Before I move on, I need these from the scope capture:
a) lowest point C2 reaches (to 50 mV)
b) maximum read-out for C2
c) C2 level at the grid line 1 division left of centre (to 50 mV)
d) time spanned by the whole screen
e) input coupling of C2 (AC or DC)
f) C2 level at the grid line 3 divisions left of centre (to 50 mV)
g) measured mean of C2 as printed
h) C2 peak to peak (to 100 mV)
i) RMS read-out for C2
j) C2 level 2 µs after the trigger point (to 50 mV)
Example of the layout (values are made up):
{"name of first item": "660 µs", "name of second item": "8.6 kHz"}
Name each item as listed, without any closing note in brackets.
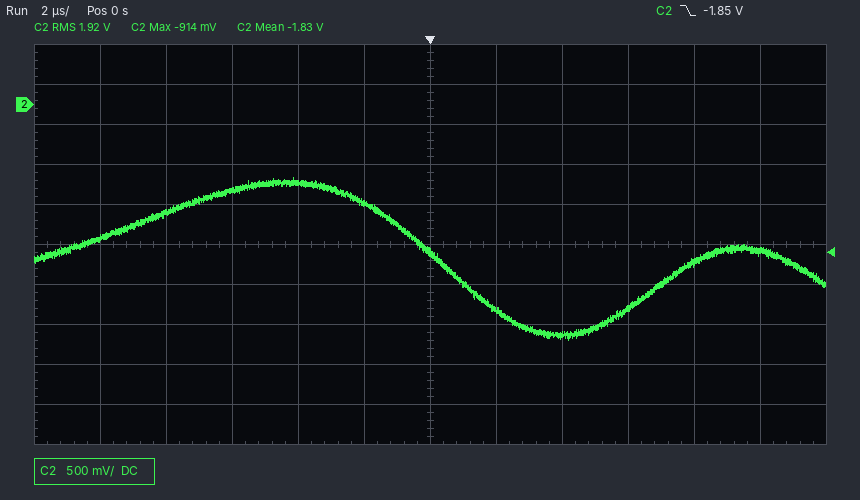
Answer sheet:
{"lowest point C2 reaches": "-2.95 V", "maximum read-out for C2": "-914 mV", "C2 level at the grid line 1 division left of centre": "-1.20 V", "time spanned by the whole screen": "24 µs", "input coupling of C2": "DC", "C2 level at the grid line 3 divisions left of centre": "-1.05 V", "measured mean of C2 as printed": "-1.83 V", "C2 peak to peak": "2.00 V", "RMS read-out for C2": "1.92 V", "C2 level 2 µs after the trigger point": "-2.55 V"}
